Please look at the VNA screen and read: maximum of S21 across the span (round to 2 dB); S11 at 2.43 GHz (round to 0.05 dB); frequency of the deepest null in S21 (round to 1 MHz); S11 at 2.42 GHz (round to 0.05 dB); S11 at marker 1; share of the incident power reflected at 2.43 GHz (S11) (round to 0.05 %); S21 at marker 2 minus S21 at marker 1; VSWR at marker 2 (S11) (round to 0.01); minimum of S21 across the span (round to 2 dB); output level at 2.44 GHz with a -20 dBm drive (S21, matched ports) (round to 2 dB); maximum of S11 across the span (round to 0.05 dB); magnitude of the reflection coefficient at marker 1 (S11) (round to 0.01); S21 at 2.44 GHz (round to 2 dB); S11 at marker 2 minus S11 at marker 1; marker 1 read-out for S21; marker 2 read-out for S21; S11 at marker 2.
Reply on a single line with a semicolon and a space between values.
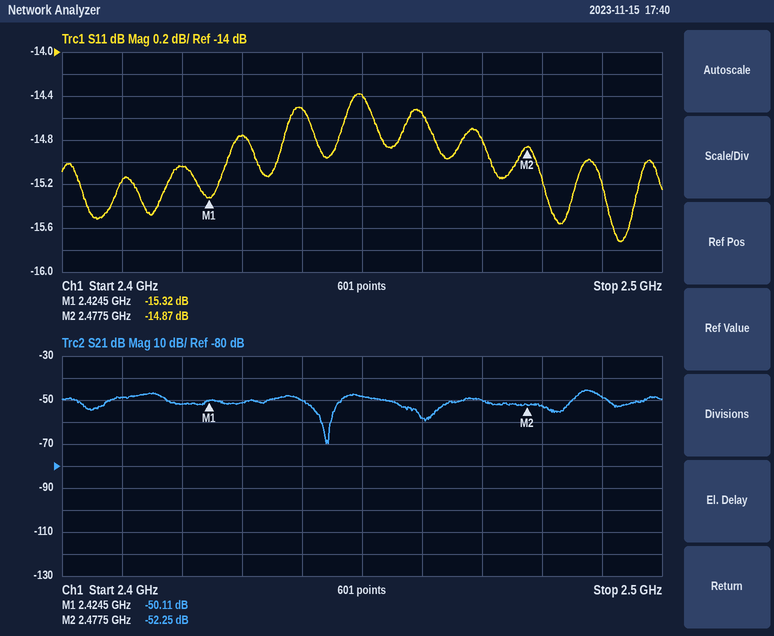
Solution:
-46 dB; -14.75 dB; 2.444 GHz; -15.05 dB; -15.32 dB; 3.35 %; -2.14 dB; 1.44; -70 dB; -70 dBm; -14.40 dB; 0.17; -50 dB; 0.45 dB; -50.11 dB; -52.25 dB; -14.87 dB
